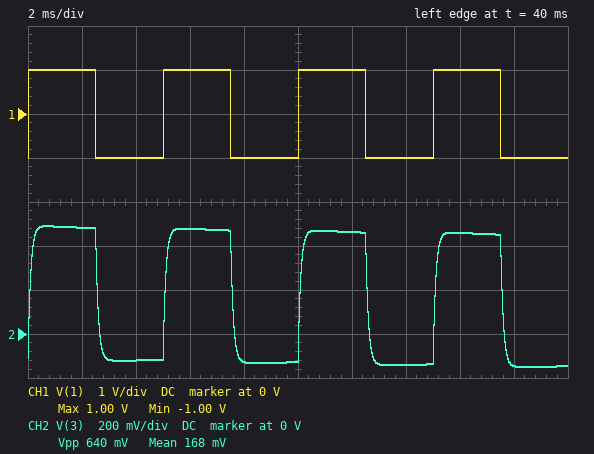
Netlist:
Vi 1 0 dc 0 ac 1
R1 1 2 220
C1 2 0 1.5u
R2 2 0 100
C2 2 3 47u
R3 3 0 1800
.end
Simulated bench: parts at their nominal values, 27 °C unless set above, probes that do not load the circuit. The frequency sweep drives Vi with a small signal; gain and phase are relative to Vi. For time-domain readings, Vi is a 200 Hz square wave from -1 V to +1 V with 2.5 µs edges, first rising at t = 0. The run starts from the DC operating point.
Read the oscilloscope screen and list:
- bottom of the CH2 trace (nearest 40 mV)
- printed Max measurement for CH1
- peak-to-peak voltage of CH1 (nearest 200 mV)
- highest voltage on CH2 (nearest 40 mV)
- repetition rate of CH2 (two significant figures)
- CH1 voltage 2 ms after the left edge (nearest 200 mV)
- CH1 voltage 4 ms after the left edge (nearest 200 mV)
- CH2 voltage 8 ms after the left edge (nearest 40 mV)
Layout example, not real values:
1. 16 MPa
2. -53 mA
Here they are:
1. -160 mV
2. 1.00 V
3. 2.0 V
4. 480 mV
5. 200 Hz
6. 1.0 V
7. -1.0 V
8. -120 mV
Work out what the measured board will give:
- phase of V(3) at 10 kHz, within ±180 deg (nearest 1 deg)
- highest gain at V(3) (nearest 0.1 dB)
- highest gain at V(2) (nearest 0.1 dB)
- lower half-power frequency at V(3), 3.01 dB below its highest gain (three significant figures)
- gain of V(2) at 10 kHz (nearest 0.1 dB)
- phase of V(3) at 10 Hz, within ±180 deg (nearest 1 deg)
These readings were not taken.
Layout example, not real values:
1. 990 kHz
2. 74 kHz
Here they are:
1. -81 deg
2. -10.4 dB
3. -10.1 dB
4. 1.81 Hz
5. -26.4 dB
6. 10 deg
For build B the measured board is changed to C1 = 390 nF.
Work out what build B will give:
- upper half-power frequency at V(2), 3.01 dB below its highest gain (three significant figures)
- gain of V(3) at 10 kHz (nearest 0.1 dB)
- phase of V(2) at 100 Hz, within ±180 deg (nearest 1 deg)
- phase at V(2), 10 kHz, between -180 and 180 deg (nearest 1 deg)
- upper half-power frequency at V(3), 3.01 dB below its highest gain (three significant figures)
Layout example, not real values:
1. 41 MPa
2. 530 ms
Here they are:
1. 5.70 kHz
2. -16.0 dB
3. -1 deg
4. -58 deg
5. 6.17 kHz
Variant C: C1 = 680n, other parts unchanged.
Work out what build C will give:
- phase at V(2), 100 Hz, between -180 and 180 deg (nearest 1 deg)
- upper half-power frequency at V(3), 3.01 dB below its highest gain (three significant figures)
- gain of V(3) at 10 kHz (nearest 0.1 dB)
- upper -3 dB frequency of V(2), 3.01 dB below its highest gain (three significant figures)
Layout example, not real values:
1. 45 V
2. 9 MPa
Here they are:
1. -2 deg
2. 3.54 kHz
3. -20.0 dB
4. 3.27 kHz
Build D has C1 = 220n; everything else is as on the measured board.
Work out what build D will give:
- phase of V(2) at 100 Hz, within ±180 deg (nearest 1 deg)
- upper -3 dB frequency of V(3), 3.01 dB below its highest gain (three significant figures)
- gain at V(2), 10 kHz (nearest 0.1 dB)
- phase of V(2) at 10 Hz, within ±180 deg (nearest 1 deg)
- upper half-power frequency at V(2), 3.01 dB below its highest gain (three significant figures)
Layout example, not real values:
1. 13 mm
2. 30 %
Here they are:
1. -1 deg
2. 10.9 kHz
3. -13.1 dB
4. 0 deg
5. 10.1 kHz
